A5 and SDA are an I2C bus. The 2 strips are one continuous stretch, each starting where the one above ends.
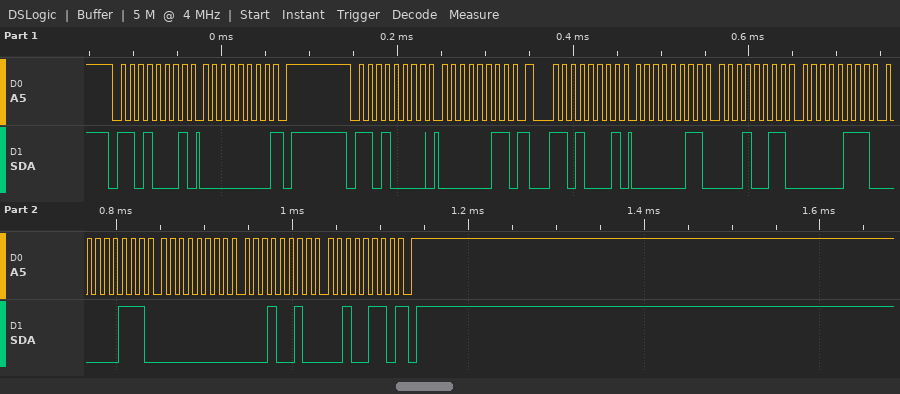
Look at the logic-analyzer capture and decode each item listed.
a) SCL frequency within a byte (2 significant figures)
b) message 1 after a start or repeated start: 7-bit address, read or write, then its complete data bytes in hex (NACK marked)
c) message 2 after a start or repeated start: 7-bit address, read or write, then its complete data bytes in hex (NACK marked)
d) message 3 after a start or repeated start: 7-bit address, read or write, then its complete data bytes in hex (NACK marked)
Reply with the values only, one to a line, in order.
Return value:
100 kHz
0x68 read: 00 NACK
0x68 write: 03
0x68 read: 03 13 07 07 00 12 26 NACK
